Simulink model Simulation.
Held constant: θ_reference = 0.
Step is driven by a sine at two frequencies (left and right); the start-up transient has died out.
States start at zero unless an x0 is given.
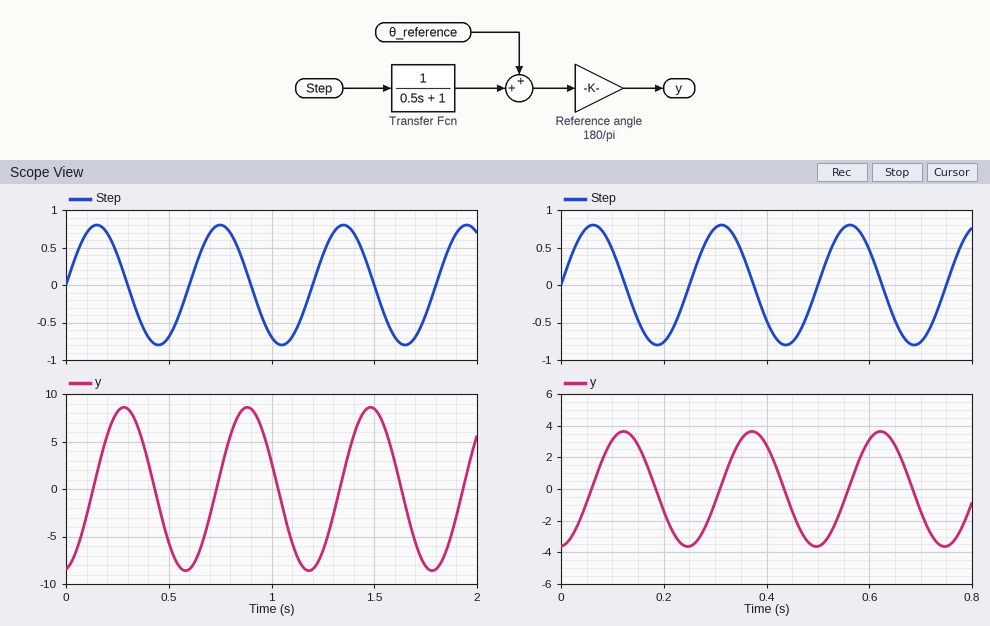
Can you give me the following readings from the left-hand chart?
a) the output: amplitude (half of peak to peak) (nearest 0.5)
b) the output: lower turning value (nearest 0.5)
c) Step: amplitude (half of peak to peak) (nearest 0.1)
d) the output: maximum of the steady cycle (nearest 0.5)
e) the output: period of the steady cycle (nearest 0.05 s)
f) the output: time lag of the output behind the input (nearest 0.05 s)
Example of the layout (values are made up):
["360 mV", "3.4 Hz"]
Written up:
["8.5", "-8.5", "0.8", "8.5", "0.60 s", "0.15 s"]
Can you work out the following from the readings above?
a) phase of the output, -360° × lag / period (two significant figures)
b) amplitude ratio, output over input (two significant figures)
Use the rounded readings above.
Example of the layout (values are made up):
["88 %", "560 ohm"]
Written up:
["-90°", "11"]
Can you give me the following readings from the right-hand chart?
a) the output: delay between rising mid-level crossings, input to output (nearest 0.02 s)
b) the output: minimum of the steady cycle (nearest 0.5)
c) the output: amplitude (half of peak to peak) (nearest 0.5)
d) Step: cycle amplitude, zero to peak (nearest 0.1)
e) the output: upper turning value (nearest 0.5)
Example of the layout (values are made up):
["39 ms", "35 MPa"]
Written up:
["0.06 s", "-3.5", "3.5", "0.8", "3.5"]
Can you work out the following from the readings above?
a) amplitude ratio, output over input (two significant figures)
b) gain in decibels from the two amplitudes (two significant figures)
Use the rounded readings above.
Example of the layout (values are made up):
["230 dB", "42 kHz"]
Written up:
["4.4", "13 dB"]
